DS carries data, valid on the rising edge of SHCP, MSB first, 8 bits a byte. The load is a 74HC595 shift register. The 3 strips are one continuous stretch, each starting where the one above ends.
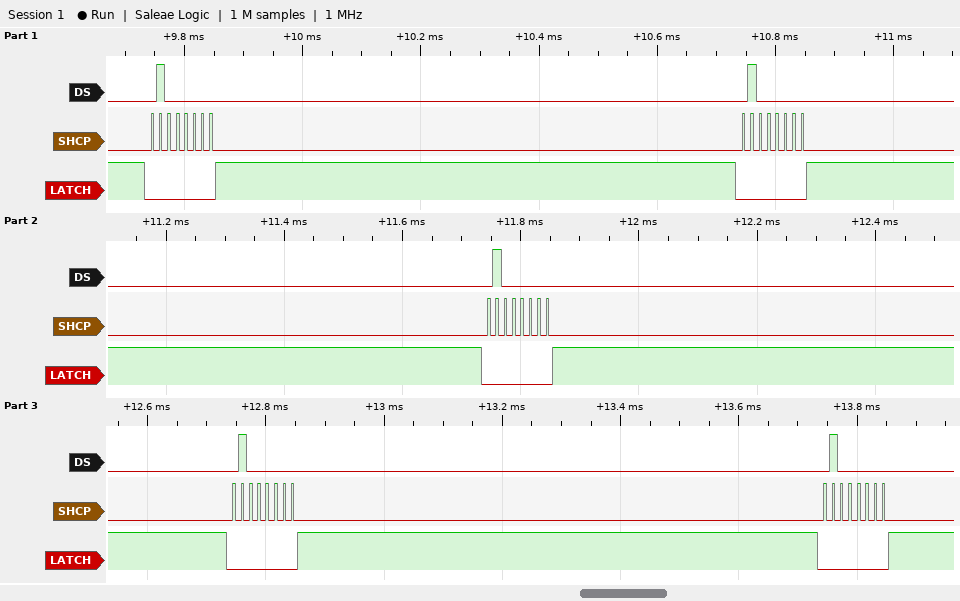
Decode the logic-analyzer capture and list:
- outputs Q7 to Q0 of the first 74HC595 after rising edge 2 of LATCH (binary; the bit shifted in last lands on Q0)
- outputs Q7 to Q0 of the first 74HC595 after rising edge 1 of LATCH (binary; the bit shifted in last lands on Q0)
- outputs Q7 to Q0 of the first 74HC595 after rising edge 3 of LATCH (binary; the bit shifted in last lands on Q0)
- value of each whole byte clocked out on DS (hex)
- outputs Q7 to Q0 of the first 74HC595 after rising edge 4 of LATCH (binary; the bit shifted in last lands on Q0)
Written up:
01000000
01000000
01000000
40 40 40 40 40
01000000
